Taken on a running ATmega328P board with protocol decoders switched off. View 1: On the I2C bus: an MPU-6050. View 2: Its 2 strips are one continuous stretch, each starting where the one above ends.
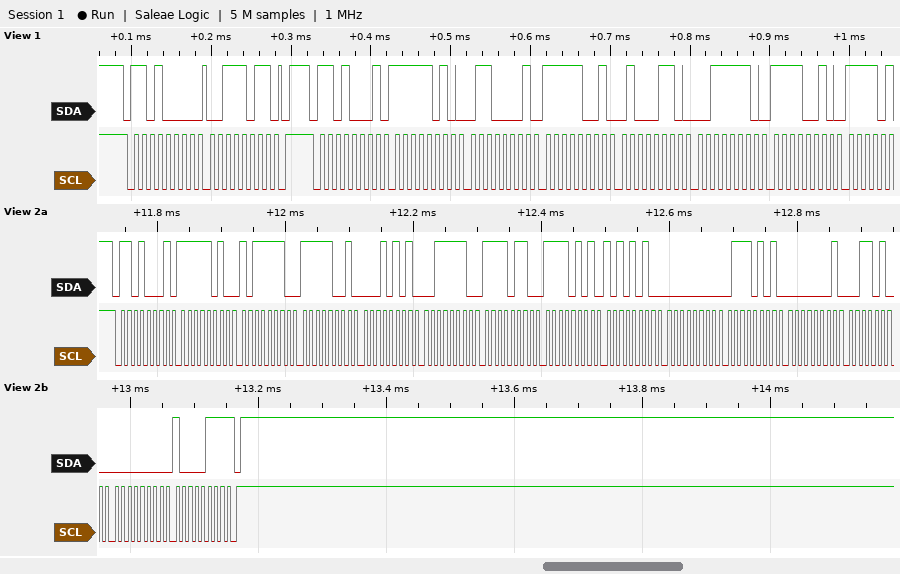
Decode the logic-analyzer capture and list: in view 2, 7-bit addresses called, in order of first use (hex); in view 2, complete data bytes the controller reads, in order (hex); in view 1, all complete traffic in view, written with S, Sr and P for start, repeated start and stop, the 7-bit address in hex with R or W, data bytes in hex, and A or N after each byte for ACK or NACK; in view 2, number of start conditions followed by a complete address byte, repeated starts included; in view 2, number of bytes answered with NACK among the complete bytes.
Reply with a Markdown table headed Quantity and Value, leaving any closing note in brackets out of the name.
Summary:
| Quantity | Value |
|---|---|
| in view 2, 7-bit addresses called, in order of first use | 0x68 |
| in view 2, complete data bytes the controller reads, in order | FA BE F9 15 3E F6 F5 AA 00 75 01 34 00 87 |
| in view 1, all complete traffic in view, written with S, Sr and P for start, repeated start and stop, the 7-bit address in hex with R or W, data bytes in hex, and A or N after each byte for ACK or NACK | S 68W A 3B A P S 68R A FA A 61 A F9 A 46 A 3E A F2 A |
| in view 2, number of start conditions followed by a complete address byte, repeated starts included | 1 |
| in view 2, number of bytes answered with NACK among the complete bytes | 1 |
